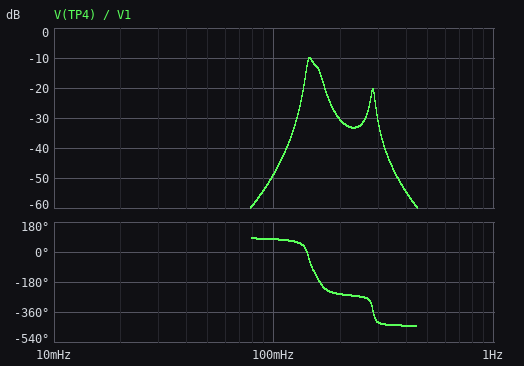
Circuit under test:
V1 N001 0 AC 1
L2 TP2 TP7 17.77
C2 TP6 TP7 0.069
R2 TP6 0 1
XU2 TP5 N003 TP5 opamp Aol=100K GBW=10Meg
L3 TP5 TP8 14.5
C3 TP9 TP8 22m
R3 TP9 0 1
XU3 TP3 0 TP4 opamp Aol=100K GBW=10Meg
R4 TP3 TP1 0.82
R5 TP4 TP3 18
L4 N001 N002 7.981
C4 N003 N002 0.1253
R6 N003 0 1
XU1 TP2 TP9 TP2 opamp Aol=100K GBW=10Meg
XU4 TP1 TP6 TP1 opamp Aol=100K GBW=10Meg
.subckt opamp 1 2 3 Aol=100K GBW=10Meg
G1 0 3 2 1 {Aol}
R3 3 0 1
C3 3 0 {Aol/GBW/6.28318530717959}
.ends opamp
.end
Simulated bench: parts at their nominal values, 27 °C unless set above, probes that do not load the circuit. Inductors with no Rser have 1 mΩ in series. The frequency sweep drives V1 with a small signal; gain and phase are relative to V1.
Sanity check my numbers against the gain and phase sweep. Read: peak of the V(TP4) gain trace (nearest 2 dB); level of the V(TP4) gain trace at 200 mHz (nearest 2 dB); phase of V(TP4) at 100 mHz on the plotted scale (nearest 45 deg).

-10 dB
-30 dB
90 deg
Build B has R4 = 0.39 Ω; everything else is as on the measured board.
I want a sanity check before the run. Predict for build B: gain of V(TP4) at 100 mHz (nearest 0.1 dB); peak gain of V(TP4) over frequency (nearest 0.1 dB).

-42.1 dB
-3.4 dB
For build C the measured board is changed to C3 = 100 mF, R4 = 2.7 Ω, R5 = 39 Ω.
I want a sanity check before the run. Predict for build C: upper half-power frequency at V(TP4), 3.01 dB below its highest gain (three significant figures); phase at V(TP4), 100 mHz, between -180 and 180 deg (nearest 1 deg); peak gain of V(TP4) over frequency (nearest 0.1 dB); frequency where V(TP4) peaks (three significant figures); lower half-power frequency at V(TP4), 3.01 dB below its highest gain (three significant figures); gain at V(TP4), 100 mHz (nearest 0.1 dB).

148 mHz
69 deg
10.5 dB
143 mHz
138 mHz
-32.9 dB
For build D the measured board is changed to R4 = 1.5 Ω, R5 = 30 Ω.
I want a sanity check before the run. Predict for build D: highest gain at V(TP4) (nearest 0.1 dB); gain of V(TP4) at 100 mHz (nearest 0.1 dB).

-10.7 dB
-49.3 dB
